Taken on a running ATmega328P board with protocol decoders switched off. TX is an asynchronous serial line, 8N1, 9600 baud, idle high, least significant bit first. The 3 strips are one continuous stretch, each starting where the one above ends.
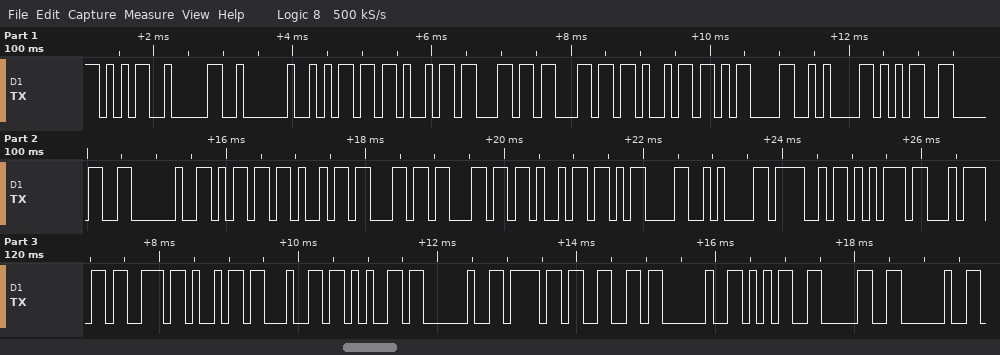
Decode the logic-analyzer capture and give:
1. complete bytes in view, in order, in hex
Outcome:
35 30 20 6D 69 6C 6C 69 0D 0A 35 30 20 6D 69 6C 6C 69 0D 0A 4F 75 74 73 69 64 65 20 6F 66 20 35 30 20
